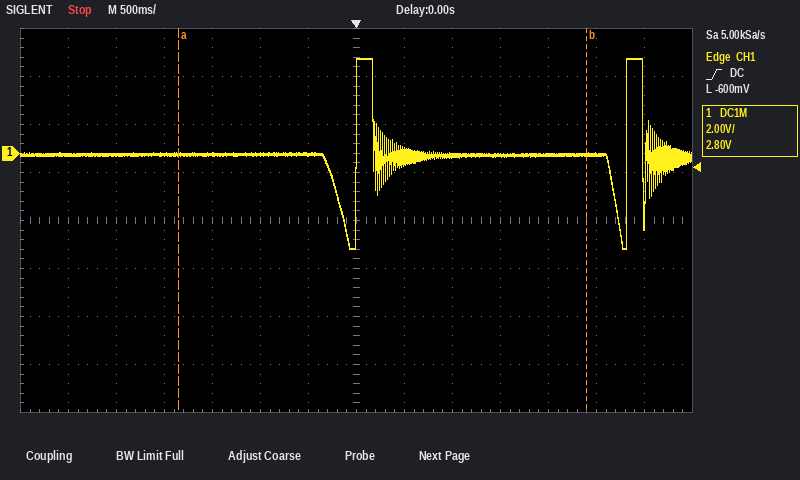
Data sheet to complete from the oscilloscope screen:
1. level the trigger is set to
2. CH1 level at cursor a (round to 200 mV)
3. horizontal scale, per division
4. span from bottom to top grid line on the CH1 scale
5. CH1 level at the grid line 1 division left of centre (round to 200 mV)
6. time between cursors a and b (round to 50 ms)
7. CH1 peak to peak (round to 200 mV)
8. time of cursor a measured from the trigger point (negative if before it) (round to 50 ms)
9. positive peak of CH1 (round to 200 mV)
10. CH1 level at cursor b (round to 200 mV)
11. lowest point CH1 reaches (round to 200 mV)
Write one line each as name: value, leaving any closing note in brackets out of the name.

level the trigger is set to: -600 mV
CH1 level at cursor a: 0.0 V
horizontal scale, per division: 500 ms
span from bottom to top grid line on the CH1 scale: 16 V
CH1 level at the grid line 1 division left of centre: 0.0 V
time between cursors a and b: 4.25 s
CH1 peak to peak: 8.0 V
time of cursor a measured from the trigger point (negative if before it): -1.85 s
positive peak of CH1: 4.0 V
CH1 level at cursor b: 0.0 V
lowest point CH1 reaches: -4.0 V
